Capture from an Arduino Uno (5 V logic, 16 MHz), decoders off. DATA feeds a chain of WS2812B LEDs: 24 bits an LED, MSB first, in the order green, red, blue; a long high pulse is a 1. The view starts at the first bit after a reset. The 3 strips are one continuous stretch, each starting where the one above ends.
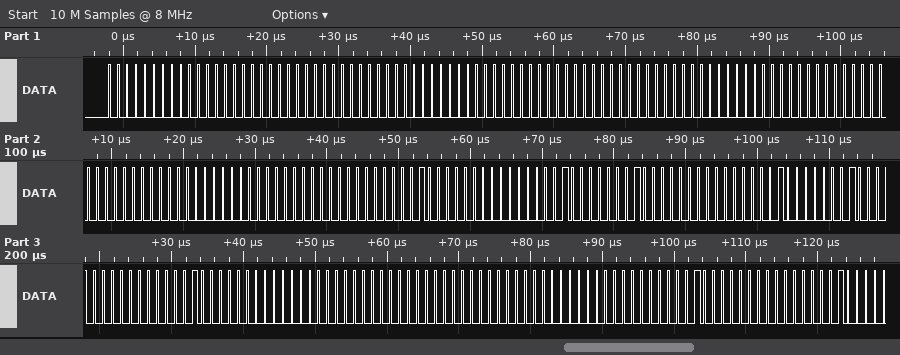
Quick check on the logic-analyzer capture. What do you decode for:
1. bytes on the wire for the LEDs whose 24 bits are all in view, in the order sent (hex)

00 00 00 00 00 00 00 00 00 00 00 00 00 00 00 08 00 08 08 00 08 08 00 08 00 00 00 00 00 00 08 00 08
